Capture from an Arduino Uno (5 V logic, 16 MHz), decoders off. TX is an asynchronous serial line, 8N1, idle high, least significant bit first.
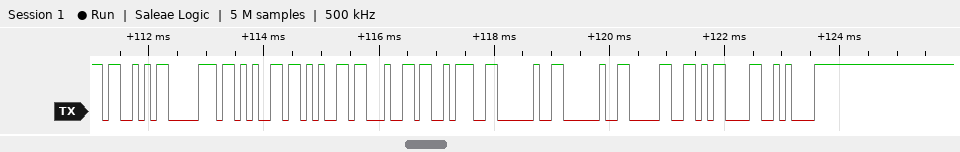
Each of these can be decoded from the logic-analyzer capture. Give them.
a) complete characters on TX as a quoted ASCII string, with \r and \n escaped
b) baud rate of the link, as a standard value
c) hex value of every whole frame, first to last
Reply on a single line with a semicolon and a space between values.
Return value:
"Speed:  0\r\n"; 9600 baud; 53 70 65 65 64 3A 20 20 30 0D 0A
